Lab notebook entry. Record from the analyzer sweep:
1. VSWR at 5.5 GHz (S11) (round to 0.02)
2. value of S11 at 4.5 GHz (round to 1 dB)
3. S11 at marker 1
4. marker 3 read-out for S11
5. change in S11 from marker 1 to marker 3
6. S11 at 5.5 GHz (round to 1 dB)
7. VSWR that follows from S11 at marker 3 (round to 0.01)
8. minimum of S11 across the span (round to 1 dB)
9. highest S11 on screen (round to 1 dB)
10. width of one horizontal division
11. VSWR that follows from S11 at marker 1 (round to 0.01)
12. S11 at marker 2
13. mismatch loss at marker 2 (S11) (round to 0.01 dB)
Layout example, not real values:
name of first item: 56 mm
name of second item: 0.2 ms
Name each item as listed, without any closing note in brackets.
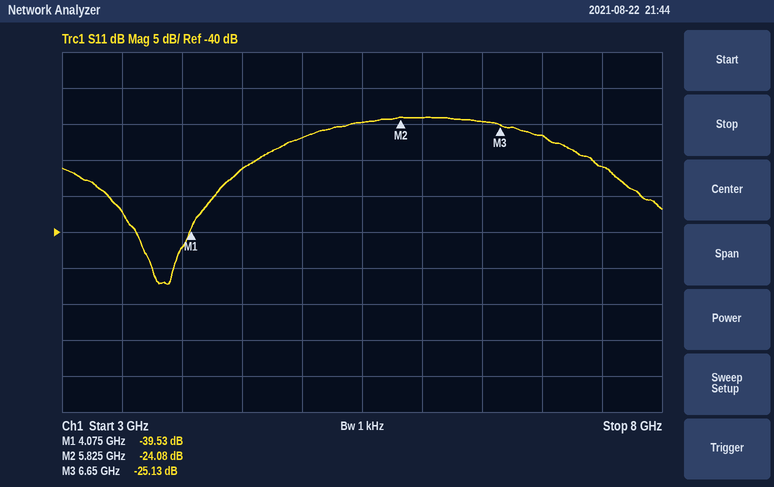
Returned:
VSWR at 5.5 GHz (S11): 1.12
value of S11 at 4.5 GHz: -31 dB
S11 at marker 1: -39.53 dB
marker 3 read-out for S11: -25.13 dB
change in S11 from marker 1 to marker 3: 14.40 dB
S11 at 5.5 GHz: -25 dB
VSWR that follows from S11 at marker 3: 1.12
minimum of S11 across the span: -47 dB
highest S11 on screen: -24 dB
width of one horizontal division: 500 MHz
VSWR that follows from S11 at marker 1: 1.02
S11 at marker 2: -24.08 dB
mismatch loss at marker 2 (S11): 0.02 dB
